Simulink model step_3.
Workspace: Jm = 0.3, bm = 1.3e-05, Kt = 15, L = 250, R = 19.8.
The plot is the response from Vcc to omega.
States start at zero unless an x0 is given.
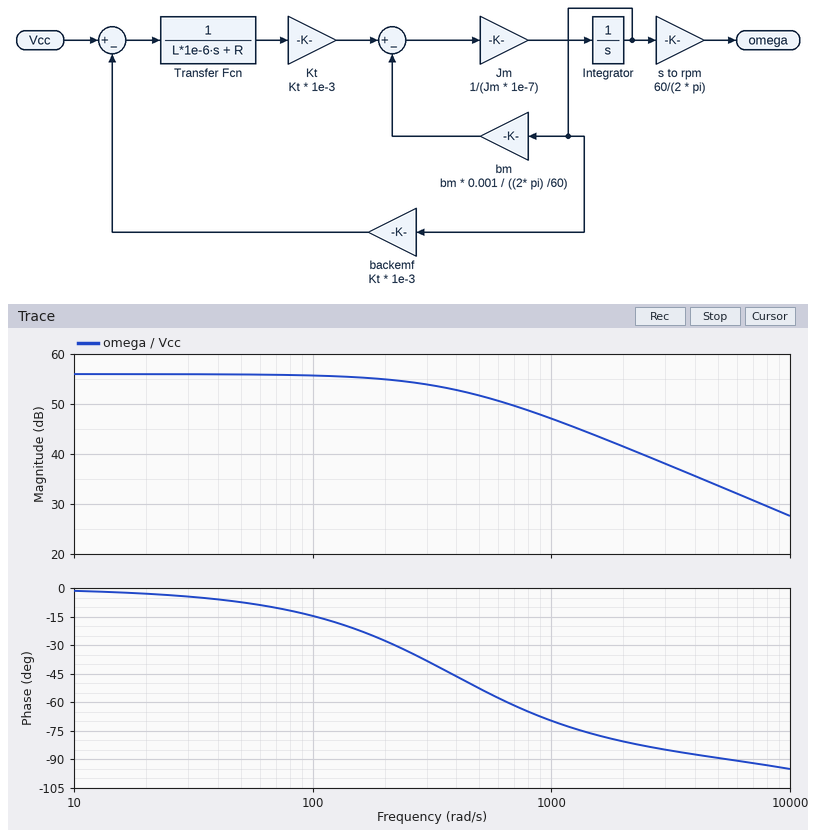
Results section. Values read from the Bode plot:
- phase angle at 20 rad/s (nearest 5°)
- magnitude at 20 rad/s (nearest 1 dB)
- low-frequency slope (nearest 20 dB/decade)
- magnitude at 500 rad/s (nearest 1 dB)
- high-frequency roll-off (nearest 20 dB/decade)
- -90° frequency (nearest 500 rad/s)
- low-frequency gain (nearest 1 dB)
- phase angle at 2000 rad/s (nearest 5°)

-5°
56 dB
0 dB/decade
52 dB
-20 dB/decade
5500 rad/s
56 dB
-80°
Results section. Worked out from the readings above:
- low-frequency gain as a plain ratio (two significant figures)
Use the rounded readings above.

630
